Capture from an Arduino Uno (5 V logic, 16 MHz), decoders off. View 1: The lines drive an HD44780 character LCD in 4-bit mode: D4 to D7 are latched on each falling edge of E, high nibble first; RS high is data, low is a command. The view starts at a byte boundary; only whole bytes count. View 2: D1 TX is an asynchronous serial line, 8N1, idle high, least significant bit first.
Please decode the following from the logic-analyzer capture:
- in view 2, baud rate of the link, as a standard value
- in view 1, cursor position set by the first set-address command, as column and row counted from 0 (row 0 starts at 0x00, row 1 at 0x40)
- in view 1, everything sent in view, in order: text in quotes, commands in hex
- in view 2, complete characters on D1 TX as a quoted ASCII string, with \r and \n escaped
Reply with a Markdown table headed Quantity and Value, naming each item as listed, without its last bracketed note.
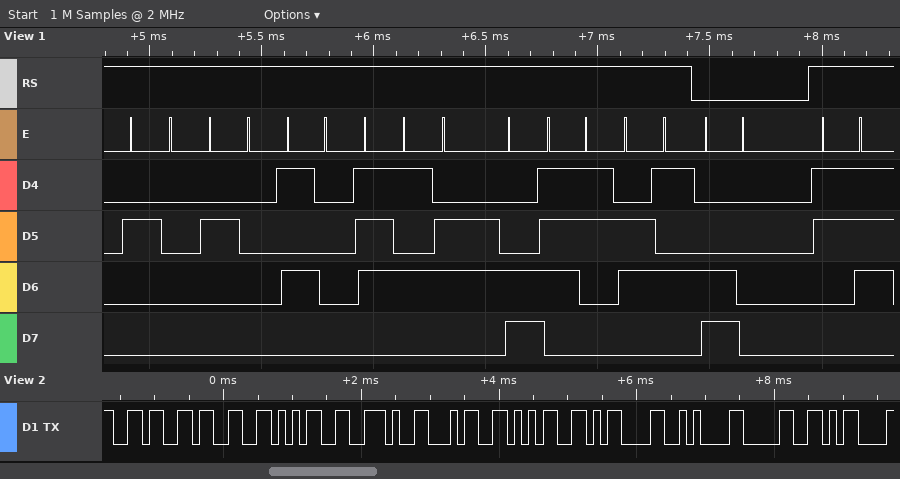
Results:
| Quantity | Value |
|---|---|
| in view 2, baud rate of the link, as a standard value | 9600 baud |
| in view 1, cursor position set by the first set-address command, as column and row counted from 0 | column 0, row 1 |
| in view 1, everything sent in view, in order: text in quotes, commands in hex | "  Pulse" 0xC0 "7" |
| in view 2, complete characters on D1 TX as a quoted ASCII string, with \r and \n escaped | "635.45\r\n0\r" |
